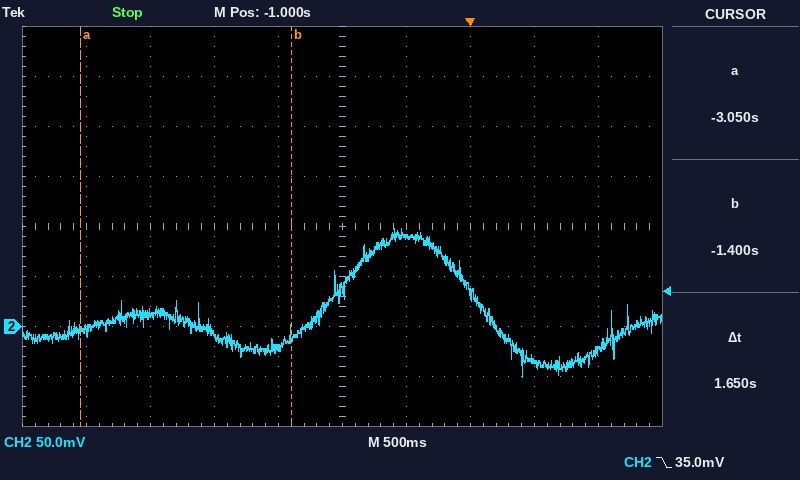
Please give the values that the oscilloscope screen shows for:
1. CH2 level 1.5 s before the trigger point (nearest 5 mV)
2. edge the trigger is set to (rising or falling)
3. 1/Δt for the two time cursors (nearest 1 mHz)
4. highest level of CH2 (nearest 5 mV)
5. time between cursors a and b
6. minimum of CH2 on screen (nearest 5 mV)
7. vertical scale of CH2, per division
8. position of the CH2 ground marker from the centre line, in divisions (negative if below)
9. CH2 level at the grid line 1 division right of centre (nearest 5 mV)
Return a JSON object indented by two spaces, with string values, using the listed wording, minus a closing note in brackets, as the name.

{
  "CH2 level 1.5 s before the trigger point": "-20 mV",
  "edge the trigger is set to": "falling",
  "1/Δt for the two time cursors": "606 mHz",
  "highest level of CH2": "100 mV",
  "time between cursors a and b": "1.65 s",
  "minimum of CH2 on screen": "-50 mV",
  "vertical scale of CH2, per division": "50 mV",
  "position of the CH2 ground marker from the centre line, in divisions": "-2.0 div",
  "CH2 level at the grid line 1 division right of centre": "90 mV"
}
